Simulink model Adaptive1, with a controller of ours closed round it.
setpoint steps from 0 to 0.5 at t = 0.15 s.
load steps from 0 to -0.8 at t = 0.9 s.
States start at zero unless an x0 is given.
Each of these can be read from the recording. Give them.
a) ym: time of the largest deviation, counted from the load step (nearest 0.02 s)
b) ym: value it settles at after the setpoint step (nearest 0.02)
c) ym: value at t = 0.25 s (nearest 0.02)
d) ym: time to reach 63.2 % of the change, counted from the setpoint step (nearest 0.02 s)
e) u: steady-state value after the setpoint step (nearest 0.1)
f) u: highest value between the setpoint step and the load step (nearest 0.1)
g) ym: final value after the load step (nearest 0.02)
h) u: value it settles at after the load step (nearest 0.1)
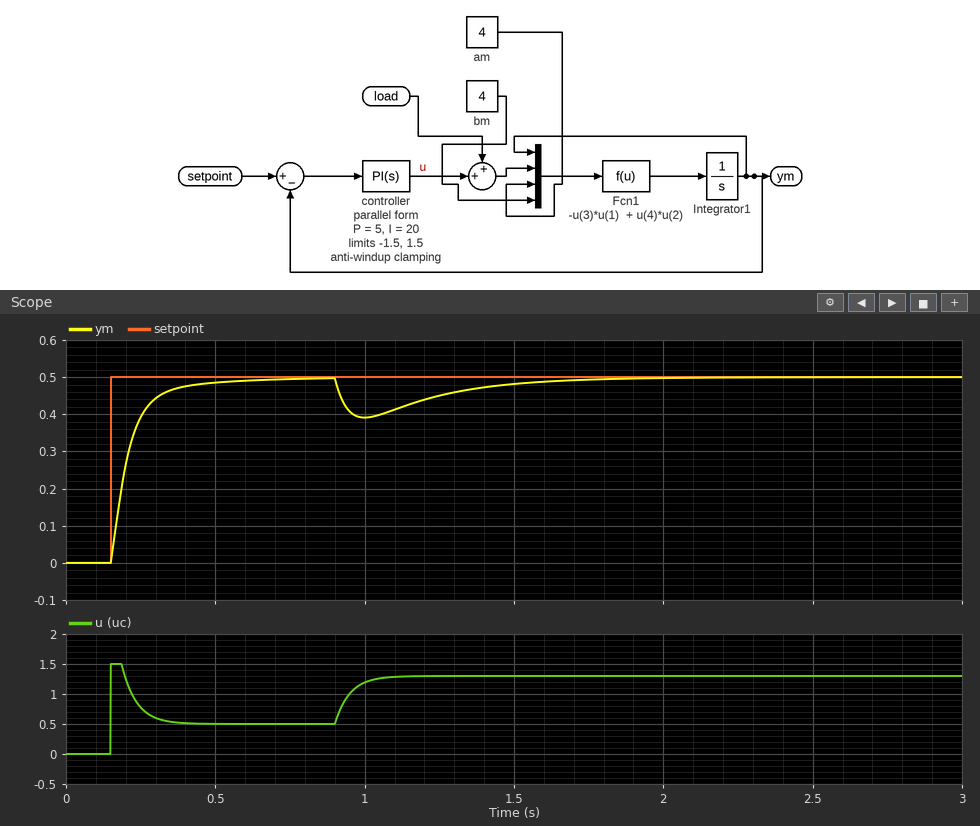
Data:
0.10 s
0.50
0.40
0.06 s
0.5
1.5
0.50
1.3
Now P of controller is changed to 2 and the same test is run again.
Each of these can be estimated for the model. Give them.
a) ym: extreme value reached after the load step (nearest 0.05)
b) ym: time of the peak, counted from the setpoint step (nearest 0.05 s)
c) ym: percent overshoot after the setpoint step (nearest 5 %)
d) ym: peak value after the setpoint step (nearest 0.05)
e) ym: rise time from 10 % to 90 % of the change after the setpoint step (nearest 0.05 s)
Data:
0.35
0.30 s
10 %
0.55
0.15 s
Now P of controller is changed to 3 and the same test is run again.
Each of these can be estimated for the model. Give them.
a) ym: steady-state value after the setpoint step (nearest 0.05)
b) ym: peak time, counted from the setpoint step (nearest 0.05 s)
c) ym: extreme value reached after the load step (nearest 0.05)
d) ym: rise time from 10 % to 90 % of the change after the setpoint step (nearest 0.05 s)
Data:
0.50
0.30 s
0.35
0.15 s
